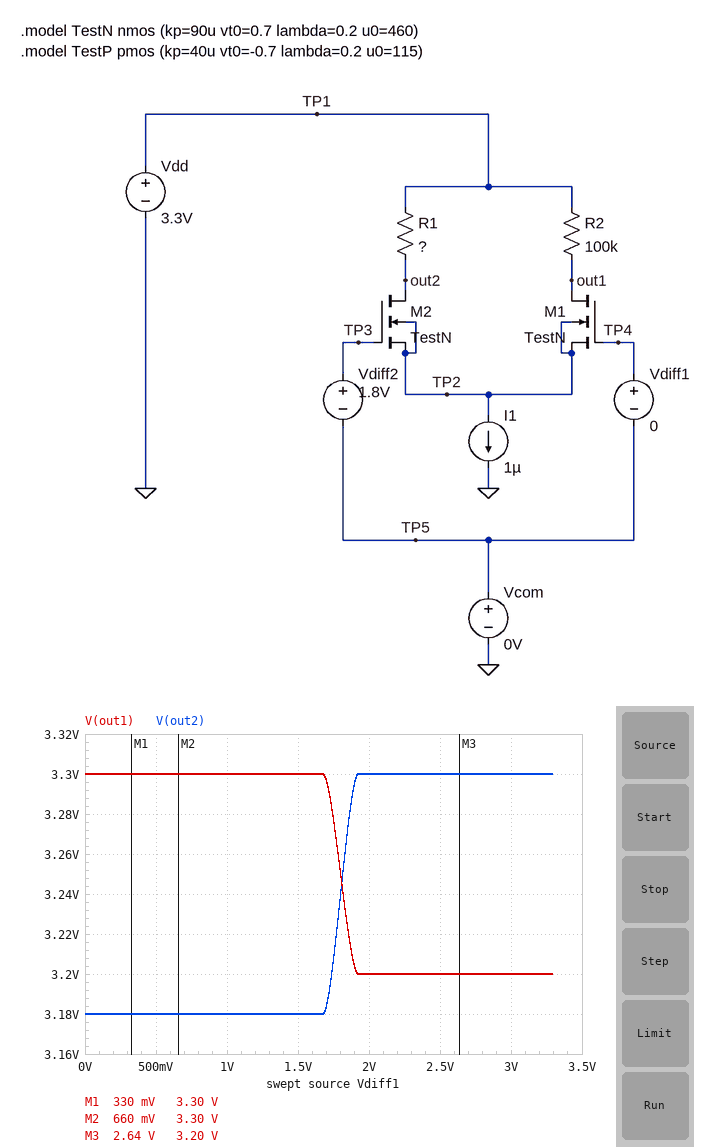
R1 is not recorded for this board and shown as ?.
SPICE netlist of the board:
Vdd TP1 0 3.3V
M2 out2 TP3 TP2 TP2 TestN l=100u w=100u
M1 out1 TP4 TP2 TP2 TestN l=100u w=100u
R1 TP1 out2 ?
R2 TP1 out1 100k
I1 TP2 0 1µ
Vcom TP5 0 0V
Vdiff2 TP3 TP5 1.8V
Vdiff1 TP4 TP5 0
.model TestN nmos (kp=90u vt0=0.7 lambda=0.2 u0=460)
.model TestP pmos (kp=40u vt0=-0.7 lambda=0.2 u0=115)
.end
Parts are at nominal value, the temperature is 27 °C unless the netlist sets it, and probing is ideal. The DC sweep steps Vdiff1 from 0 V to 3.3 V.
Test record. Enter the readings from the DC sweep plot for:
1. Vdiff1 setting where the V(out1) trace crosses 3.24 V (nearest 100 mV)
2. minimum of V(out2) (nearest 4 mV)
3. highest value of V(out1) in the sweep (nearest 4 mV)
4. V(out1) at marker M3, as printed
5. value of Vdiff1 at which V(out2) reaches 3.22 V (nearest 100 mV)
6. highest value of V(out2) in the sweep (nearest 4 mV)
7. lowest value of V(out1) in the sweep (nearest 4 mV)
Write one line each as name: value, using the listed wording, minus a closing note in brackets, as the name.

Vdiff1 setting where the V(out1) trace crosses 3.24 V: 1.8 V
minimum of V(out2): 3.180 V
highest value of V(out1) in the sweep: 3.300 V
V(out1) at marker M3, as printed: 3.20 V
value of Vdiff1 at which V(out2) reaches 3.22 V: 1.8 V
highest value of V(out2) in the sweep: 3.300 V
lowest value of V(out1) in the sweep: 3.200 V
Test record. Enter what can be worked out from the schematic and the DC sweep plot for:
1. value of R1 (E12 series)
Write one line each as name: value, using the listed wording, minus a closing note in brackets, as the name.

value of R1: 120 kΩ
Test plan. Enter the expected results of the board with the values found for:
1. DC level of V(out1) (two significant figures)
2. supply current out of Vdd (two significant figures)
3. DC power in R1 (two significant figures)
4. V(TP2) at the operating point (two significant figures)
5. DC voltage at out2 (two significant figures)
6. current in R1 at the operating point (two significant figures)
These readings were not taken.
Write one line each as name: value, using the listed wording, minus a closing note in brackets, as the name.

DC level of V(out1): 3.3 V
supply current out of Vdd: 1.0 µA
DC power in R1: 120 nW
V(TP2) at the operating point: 980 mV
DC voltage at out2: 3.2 V
current in R1 at the operating point: 1.0 µA
